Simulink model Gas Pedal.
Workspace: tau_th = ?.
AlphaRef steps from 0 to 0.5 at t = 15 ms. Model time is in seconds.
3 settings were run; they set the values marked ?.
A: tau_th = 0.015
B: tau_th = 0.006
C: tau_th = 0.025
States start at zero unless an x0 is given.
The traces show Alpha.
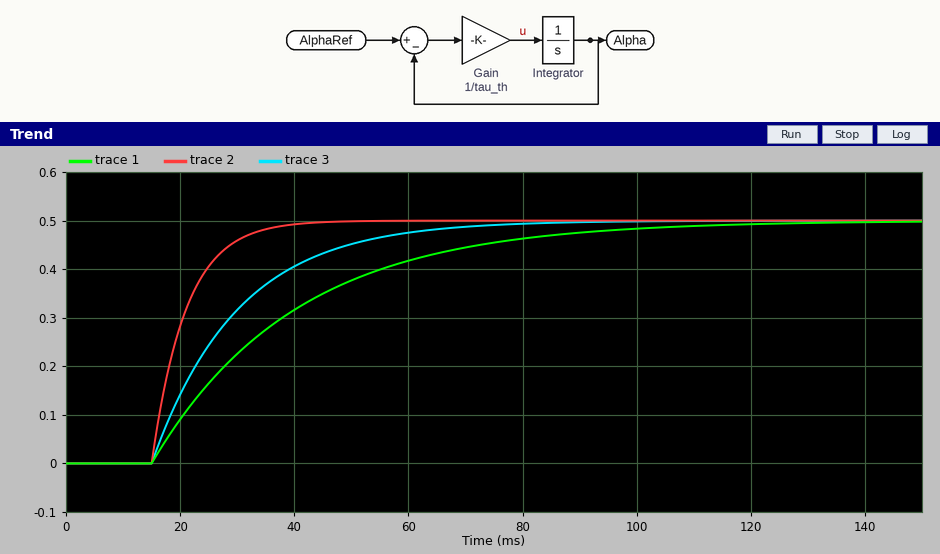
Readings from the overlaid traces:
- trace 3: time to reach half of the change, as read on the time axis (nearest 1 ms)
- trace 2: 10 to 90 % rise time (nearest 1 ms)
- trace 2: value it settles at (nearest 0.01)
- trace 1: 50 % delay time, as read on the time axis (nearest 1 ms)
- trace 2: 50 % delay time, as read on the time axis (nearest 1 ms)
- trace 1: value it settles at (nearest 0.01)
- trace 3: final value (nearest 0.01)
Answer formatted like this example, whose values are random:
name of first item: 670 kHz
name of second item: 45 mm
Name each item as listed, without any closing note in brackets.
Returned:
trace 3: time to reach half of the change, as read on the time axis: 25 ms
trace 2: 10 to 90 % rise time: 13 ms
trace 2: value it settles at: 0.50
trace 1: 50 % delay time, as read on the time axis: 32 ms
trace 2: 50 % delay time, as read on the time axis: 19 ms
trace 1: value it settles at: 0.50
trace 3: final value: 0.50
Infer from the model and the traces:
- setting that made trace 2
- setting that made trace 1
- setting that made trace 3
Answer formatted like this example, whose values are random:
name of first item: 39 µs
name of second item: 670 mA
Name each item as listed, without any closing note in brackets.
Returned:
setting that made trace 2: B
setting that made trace 1: C
setting that made trace 3: A
